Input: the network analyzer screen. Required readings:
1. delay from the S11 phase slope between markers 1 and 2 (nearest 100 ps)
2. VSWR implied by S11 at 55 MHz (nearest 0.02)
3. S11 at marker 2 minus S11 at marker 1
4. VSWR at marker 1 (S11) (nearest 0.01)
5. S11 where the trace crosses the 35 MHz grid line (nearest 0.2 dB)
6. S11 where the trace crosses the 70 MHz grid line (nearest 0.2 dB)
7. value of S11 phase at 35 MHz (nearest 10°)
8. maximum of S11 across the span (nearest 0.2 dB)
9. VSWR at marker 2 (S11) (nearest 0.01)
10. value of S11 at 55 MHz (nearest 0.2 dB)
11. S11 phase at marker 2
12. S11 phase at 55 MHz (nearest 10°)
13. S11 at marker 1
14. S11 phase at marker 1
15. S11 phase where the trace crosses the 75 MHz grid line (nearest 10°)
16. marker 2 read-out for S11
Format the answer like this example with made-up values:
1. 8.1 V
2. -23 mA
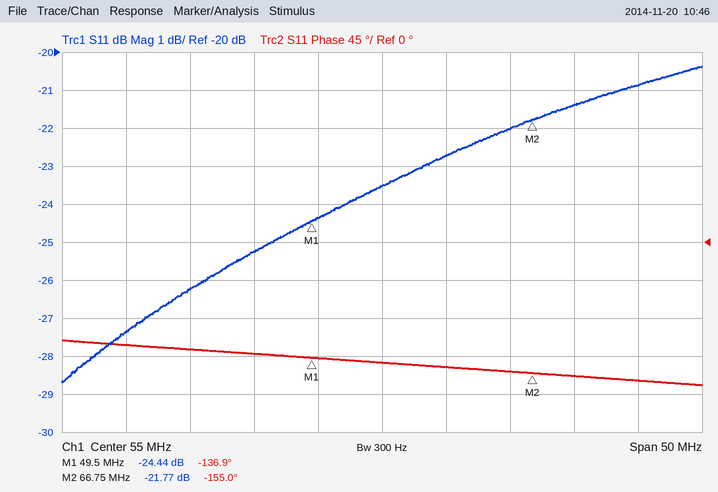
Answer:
1. 2.9 ns
2. 1.14
3. 2.67 dB
4. 1.13
5. -27.4 dB
6. -21.4 dB
7. -120°
8. -20.4 dB
9. 1.18
10. -23.6 dB
11. -155.0°
12. -140°
13. -24.44 dB
14. -136.9°
15. -160°
16. -21.77 dB
